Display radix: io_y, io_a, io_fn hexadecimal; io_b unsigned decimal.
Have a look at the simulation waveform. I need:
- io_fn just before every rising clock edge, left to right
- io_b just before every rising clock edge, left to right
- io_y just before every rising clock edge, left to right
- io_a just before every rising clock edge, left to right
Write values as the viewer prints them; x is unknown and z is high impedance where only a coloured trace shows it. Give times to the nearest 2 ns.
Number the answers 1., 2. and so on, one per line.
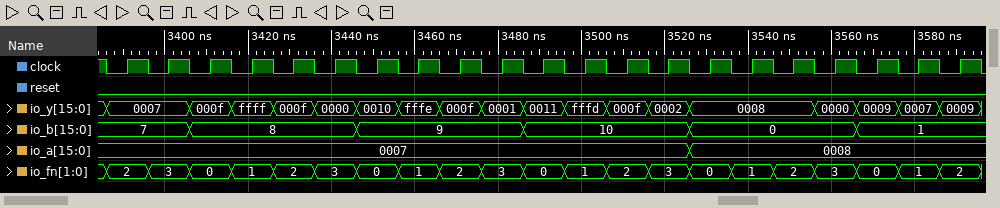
1. 2, 3, 0, 1, 2, 3, 0, 1, 2, 3, 0, 1, 2, 3, 0, 1, 2, 3, 0, 1, 2
2. 7, 7, 8, 8, 8, 8, 9, 9, 9, 9, 10, 10, 10, 10, 0, 0, 0, 0, 1, 1, 1
3. 0007, 0007, 000f, ffff, 000f, 0000, 0010, fffe, 000f, 0001, 0011, fffd, 000f, 0002, 0008, 0008, 0008, 0000, 0009, 0007, 0009
4. 0007, 0007, 0007, 0007, 0007, 0007, 0007, 0007, 0007, 0007, 0007, 0007, 0007, 0007, 0008, 0008, 0008, 0008, 0008, 0008, 0008
